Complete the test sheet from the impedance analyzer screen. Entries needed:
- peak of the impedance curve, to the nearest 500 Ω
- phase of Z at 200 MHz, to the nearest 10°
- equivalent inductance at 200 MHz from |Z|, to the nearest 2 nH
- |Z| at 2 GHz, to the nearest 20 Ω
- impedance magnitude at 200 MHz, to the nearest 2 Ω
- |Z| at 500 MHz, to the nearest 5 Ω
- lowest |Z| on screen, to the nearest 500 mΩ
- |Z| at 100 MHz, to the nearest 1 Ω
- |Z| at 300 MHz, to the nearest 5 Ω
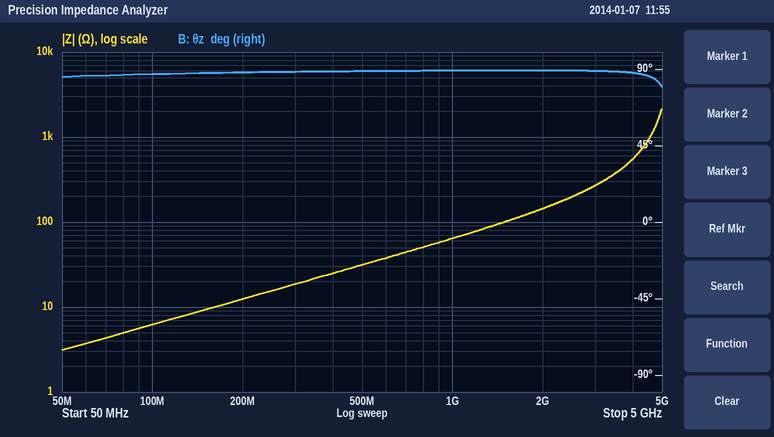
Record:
2.0 kΩ
90°
10 nH
140 Ω
12 Ω
30 Ω
3.0 Ω
6 Ω
20 Ω
